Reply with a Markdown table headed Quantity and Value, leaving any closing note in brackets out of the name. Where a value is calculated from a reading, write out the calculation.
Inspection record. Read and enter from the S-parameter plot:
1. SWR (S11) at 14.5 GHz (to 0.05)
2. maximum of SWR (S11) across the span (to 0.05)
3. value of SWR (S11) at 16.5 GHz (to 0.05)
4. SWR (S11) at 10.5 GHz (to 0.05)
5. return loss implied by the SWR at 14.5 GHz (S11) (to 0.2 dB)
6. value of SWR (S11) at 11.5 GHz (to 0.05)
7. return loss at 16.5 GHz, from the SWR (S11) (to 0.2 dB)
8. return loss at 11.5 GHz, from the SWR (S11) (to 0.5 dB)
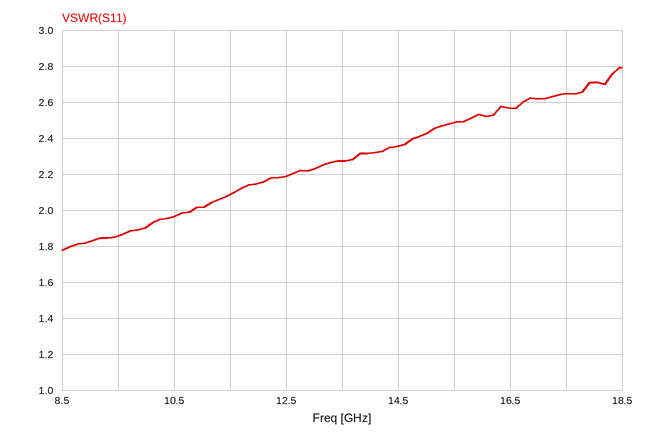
| Quantity | Value |
|---|---|
| SWR (S11) at 14.5 GHz | 2.35 |
| maximum of SWR (S11) across the span | 2.80 |
| value of SWR (S11) at 16.5 GHz | 2.55 |
| SWR (S11) at 10.5 GHz | 1.95 |
| return loss implied by the SWR at 14.5 GHz (S11) | −20 log10((2.35 − 1)/(2.35 + 1)) ≈ 7.89 dB, so 7.8 dB to the nearest 0.2 dB |
| value of SWR (S11) at 11.5 GHz | 2.10 |
| return loss at 16.5 GHz, from the SWR (S11) | −20 log10((2.55 − 1)/(2.55 + 1)) ≈ 7.2 dB |
| return loss at 11.5 GHz, from the SWR (S11) | −20 log10((2.1 − 1)/(2.1 + 1)) ≈ 9.0 dB |
